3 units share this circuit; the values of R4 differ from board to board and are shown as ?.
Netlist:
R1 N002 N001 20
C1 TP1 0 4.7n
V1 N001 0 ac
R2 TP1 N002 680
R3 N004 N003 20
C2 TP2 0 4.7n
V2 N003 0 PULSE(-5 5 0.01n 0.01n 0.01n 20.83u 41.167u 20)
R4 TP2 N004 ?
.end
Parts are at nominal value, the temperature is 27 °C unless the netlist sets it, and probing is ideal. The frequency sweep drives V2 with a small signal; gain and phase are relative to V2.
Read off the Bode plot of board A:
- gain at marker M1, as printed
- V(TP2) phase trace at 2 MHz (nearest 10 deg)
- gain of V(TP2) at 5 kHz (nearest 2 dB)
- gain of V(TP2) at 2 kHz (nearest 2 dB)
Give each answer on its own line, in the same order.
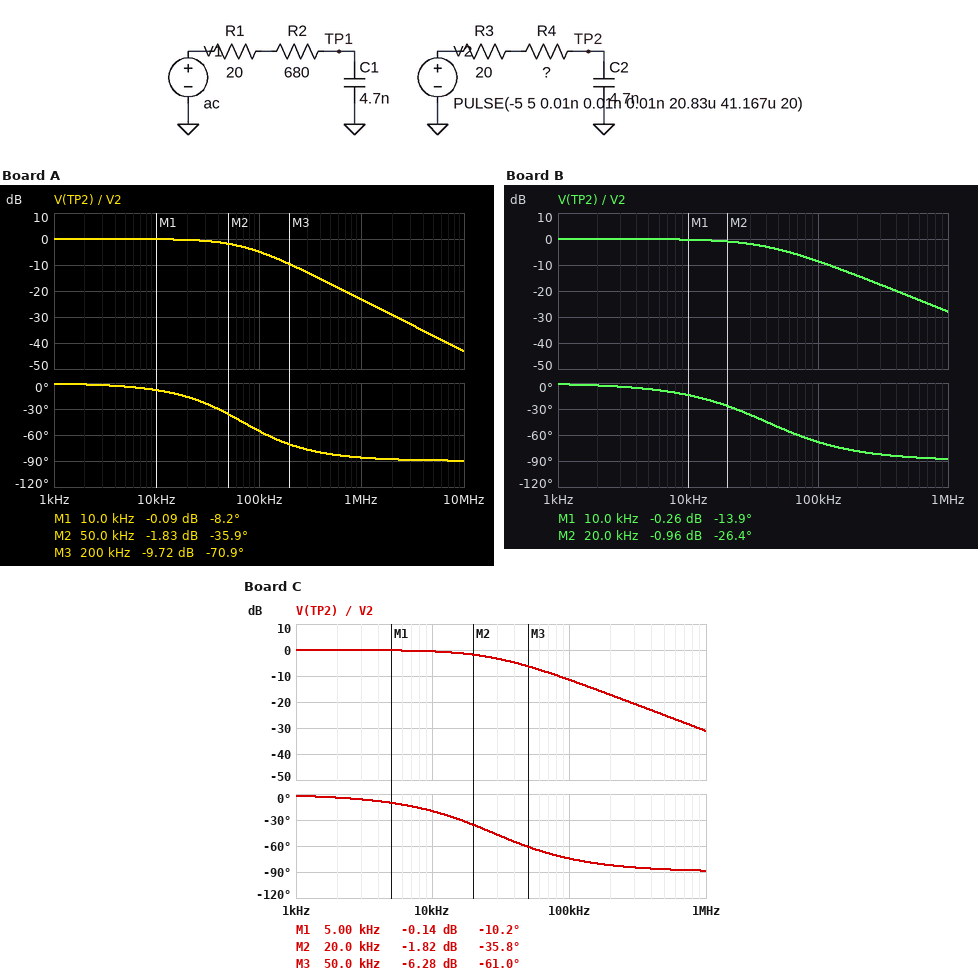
-0.09 dB
-90 deg
0 dB
0 dB
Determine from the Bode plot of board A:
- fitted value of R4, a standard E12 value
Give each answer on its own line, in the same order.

470 Ω
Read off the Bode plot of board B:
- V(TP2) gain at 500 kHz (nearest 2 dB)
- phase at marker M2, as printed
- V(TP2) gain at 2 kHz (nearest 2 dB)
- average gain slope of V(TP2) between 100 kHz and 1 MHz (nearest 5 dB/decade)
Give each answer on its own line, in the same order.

-22 dB
-26.4 deg
0 dB
-20 dB/decade
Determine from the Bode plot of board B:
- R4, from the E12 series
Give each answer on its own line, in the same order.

820 Ω
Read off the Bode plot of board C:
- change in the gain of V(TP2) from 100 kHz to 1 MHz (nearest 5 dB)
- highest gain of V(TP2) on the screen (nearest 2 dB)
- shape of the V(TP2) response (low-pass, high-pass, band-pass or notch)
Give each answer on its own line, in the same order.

-20 dB
0 dB
low-pass
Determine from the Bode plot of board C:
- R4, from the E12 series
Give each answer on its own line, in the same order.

1.2 kΩ
